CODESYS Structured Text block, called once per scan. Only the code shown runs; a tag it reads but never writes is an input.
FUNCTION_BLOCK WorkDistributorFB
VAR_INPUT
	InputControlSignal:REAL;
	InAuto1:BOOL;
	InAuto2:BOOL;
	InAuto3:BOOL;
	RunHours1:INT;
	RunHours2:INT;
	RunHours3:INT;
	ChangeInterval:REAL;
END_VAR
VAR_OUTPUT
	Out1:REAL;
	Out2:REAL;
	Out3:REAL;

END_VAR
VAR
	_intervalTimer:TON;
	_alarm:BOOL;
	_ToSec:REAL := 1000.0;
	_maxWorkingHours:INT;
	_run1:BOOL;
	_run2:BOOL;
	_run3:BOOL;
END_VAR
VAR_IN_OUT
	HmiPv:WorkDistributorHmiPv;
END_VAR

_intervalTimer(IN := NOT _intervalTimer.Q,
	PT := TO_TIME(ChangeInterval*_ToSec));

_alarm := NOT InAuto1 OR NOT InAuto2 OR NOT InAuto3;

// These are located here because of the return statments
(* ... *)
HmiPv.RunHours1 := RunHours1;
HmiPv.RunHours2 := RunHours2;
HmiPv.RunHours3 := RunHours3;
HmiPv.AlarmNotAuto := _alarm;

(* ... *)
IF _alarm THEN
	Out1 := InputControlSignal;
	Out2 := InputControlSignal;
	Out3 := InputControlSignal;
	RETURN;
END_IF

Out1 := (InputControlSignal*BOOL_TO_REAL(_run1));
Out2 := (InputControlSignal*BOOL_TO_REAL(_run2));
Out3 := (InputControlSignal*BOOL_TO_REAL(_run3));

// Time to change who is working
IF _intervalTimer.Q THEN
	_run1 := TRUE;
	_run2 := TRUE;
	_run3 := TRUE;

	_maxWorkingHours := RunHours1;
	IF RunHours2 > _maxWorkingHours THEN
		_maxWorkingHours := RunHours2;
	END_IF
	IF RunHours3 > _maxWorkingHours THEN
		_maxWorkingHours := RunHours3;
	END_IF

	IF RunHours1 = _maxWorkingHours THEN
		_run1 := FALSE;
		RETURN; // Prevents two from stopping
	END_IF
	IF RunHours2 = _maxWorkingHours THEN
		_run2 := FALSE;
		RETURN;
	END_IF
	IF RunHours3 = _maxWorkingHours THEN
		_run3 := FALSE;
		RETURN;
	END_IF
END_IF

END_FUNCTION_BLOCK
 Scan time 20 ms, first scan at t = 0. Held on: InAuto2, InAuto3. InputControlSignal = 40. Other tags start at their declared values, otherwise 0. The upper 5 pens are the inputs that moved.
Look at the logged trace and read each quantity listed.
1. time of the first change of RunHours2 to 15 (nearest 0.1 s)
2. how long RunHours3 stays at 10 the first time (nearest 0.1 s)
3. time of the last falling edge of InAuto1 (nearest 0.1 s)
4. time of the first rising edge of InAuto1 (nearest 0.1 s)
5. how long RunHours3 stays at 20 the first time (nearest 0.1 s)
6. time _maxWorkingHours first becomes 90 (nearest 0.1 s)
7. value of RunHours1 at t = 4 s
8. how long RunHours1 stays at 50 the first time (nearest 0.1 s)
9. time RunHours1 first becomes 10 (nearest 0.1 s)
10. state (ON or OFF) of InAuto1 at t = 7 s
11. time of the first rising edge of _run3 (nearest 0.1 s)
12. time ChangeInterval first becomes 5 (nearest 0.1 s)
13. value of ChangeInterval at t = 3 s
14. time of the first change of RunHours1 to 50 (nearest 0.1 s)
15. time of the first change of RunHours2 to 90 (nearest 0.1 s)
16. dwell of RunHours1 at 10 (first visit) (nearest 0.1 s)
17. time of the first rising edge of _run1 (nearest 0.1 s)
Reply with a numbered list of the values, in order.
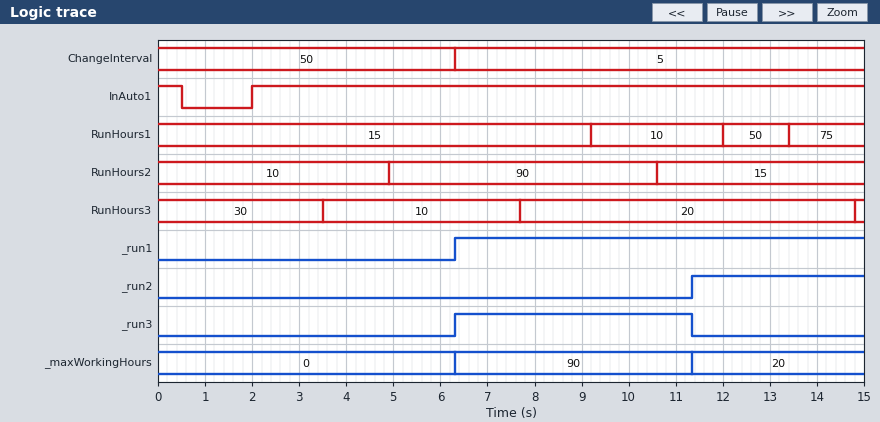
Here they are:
1. 10.6 s
2. 4.2 s
3. 0.5 s
4. 2.0 s
5. 7.1 s
6. 6.3 s
7. 15
8. 1.4 s
9. 9.2 s
10. ON
11. 6.3 s
12. 6.3 s
13. 50
14. 12.0 s
15. 4.9 s
16. 2.8 s
17. 6.3 s
